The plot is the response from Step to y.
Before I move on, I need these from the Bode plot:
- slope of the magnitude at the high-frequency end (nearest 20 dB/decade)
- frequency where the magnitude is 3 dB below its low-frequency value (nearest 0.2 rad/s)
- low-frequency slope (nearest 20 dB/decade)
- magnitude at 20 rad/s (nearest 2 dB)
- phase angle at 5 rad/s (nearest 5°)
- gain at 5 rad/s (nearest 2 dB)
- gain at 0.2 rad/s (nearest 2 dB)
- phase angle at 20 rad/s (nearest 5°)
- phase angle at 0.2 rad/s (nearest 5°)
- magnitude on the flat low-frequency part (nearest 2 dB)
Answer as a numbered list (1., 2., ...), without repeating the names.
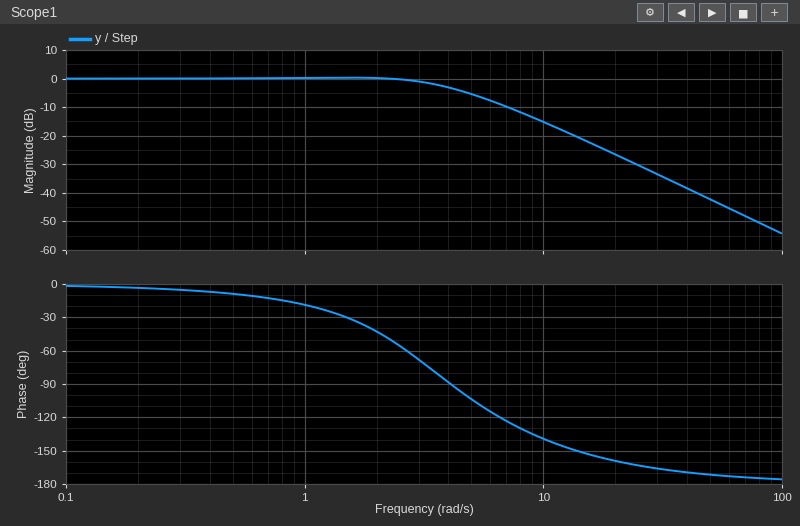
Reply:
1. -40 dB/decade
2. 4.0 rad/s
3. 0 dB/decade
4. -26 dB
5. -105°
6. -6 dB
7. 0 dB
8. -160°
9. -5°
10. 0 dB
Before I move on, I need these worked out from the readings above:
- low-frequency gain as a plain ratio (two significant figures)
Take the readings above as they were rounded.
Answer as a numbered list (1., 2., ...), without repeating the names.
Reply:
1. 1.0
